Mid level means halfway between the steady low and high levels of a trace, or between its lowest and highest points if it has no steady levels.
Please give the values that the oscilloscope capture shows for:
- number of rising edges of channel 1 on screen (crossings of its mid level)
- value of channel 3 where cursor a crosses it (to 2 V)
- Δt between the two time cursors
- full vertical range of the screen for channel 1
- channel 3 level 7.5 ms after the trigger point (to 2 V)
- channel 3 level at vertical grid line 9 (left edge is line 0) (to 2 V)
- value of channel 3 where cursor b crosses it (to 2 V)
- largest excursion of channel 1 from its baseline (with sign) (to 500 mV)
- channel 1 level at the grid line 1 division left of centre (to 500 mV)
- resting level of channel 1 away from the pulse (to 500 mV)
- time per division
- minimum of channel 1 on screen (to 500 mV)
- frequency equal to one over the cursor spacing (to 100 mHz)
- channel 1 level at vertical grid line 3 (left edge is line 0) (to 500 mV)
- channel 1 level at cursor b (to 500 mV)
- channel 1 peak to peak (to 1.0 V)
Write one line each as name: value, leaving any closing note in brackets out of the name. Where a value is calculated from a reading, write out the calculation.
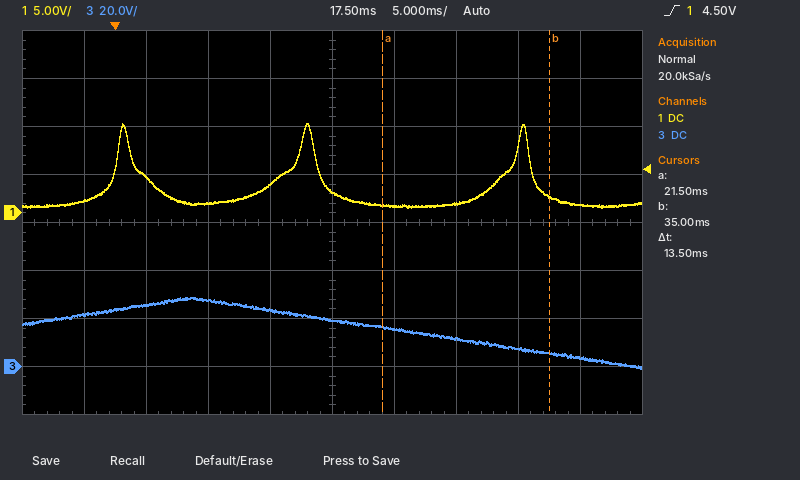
number of rising edges of channel 1 on screen: 3
value of channel 3 where cursor a crosses it: 16 V
Δt between the two time cursors: 13.5 ms
full vertical range of the screen for channel 1: 40 V
channel 3 level 7.5 ms after the trigger point: 28 V
channel 3 level at vertical grid line 9 (left edge is line 0): 4 V
value of channel 3 where cursor b crosses it: 6 V
largest excursion of channel 1 from its baseline (with sign): +8.5 V
channel 1 level at the grid line 1 division left of centre: 3.0 V
resting level of channel 1 away from the pulse: 1.0 V
time per division: 5 ms
minimum of channel 1 on screen: 500 mV
frequency equal to one over the cursor spacing: 1 / 13.5 ms ≈ 74.1 Hz
channel 1 level at vertical grid line 3 (left edge is line 0): 1.0 V
channel 1 level at cursor b: 1.5 V
channel 1 peak to peak: 9.0 V
